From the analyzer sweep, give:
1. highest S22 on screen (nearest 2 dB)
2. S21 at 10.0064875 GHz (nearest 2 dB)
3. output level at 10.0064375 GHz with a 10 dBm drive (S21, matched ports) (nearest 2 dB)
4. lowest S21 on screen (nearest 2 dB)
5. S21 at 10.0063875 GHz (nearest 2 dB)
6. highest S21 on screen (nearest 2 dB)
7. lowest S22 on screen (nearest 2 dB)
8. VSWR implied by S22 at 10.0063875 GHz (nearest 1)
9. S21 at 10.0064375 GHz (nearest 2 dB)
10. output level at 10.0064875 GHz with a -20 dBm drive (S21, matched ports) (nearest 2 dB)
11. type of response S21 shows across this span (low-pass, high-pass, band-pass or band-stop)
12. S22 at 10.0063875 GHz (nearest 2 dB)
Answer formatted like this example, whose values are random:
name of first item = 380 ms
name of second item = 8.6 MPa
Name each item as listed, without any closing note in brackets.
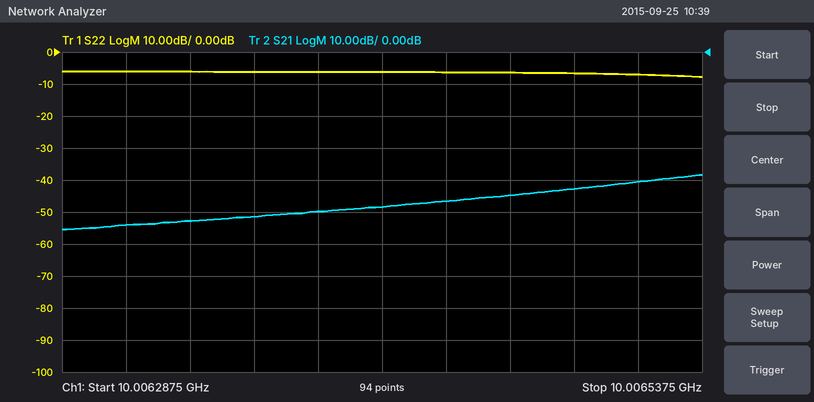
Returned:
highest S22 on screen = -6 dB
S21 at 10.0064875 GHz = -42 dB
output level at 10.0064375 GHz with a 10 dBm drive (S21, matched ports) = -36 dBm
lowest S21 on screen = -56 dB
S21 at 10.0063875 GHz = -50 dB
highest S21 on screen = -38 dB
lowest S22 on screen = -8 dB
VSWR implied by S22 at 10.0063875 GHz = 3
S21 at 10.0064375 GHz = -46 dB
output level at 10.0064875 GHz with a -20 dBm drive (S21, matched ports) = -62 dBm
type of response S21 shows across this span = high-pass
S22 at 10.0063875 GHz = -6 dB
